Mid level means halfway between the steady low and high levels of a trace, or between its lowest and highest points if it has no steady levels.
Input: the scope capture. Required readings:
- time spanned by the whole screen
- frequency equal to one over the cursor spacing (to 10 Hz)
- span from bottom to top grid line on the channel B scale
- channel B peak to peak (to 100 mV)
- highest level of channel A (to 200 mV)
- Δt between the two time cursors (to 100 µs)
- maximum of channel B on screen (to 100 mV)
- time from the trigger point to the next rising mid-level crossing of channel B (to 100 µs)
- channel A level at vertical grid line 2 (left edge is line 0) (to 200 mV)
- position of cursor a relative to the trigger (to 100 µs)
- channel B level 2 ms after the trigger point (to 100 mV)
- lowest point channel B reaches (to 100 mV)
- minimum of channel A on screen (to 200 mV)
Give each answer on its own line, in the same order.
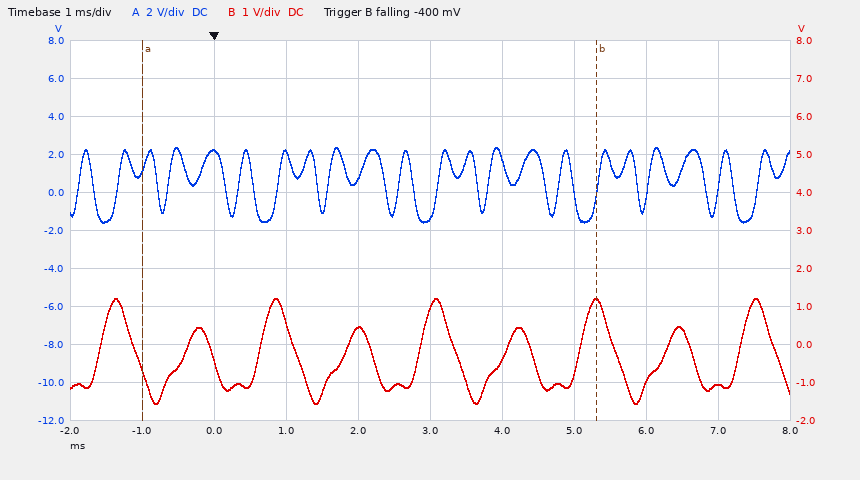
10 ms
160 Hz
10 V
2.8 V
2.4 V
6.3 ms
1.2 V
600 µs
2.2 V
-1.0 ms
400 mV
-1.6 V
-1.6 V
